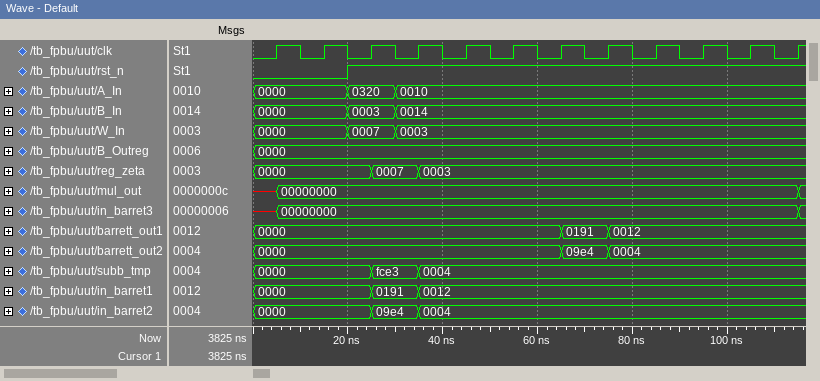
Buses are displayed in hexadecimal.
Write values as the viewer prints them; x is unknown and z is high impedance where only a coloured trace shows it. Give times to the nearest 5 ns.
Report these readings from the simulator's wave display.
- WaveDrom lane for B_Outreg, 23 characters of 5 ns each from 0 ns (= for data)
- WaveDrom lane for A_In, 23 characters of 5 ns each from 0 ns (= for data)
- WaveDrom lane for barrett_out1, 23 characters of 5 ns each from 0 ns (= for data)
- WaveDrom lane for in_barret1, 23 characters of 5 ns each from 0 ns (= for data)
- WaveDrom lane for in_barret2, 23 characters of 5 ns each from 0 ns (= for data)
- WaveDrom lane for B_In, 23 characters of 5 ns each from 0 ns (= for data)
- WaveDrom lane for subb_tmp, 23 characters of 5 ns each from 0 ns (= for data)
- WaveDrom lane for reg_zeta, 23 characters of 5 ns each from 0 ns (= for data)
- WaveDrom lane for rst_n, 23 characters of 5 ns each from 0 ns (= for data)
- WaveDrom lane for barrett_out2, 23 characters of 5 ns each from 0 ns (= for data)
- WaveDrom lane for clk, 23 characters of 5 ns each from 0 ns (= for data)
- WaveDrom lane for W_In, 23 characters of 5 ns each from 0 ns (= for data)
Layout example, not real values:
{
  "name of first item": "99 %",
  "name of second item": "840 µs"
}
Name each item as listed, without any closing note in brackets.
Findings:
{
  "WaveDrom lane for B_Outreg, 23 characters of 5 ns each from 0 ns": "{name: 'B_Outreg', wave: '=......................', data: '0000'}",
  "WaveDrom lane for A_In, 23 characters of 5 ns each from 0 ns": "{name: 'A_In', wave: '=...=.=................', data: '0000 0320 0010'}",
  "WaveDrom lane for barrett_out1, 23 characters of 5 ns each from 0 ns": "{name: 'barrett_out1', wave: '=............=.=.......', data: '0000 0191 0012'}",
  "WaveDrom lane for in_barret1, 23 characters of 5 ns each from 0 ns": "{name: 'in_barret1', wave: '=....=.=...............', data: '0000 0191 0012'}",
  "WaveDrom lane for in_barret2, 23 characters of 5 ns each from 0 ns": "{name: 'in_barret2', wave: '=....=.=...............', data: '0000 09e4 0004'}",
  "WaveDrom lane for B_In, 23 characters of 5 ns each from 0 ns": "{name: 'B_In', wave: '=...=.=................', data: '0000 0003 0014'}",
  "WaveDrom lane for subb_tmp, 23 characters of 5 ns each from 0 ns": "{name: 'subb_tmp', wave: '=....=.=...............', data: '0000 fce3 0004'}",
  "WaveDrom lane for reg_zeta, 23 characters of 5 ns each from 0 ns": "{name: 'reg_zeta', wave: '=....=.=...............', data: '0000 0007 0003'}",
  "WaveDrom lane for rst_n, 23 characters of 5 ns each from 0 ns": "{name: 'rst_n', wave: '0...1..................'}",
  "WaveDrom lane for barrett_out2, 23 characters of 5 ns each from 0 ns": "{name: 'barrett_out2', wave: '=............=.=.......', data: '0000 09e4 0004'}",
  "WaveDrom lane for clk, 23 characters of 5 ns each from 0 ns": "{name: 'clk', wave: '01010101010101010101010'}",
  "WaveDrom lane for W_In, 23 characters of 5 ns each from 0 ns": "{name: 'W_In', wave: '=...=.=................', data: '0000 0007 0003'}"
}
